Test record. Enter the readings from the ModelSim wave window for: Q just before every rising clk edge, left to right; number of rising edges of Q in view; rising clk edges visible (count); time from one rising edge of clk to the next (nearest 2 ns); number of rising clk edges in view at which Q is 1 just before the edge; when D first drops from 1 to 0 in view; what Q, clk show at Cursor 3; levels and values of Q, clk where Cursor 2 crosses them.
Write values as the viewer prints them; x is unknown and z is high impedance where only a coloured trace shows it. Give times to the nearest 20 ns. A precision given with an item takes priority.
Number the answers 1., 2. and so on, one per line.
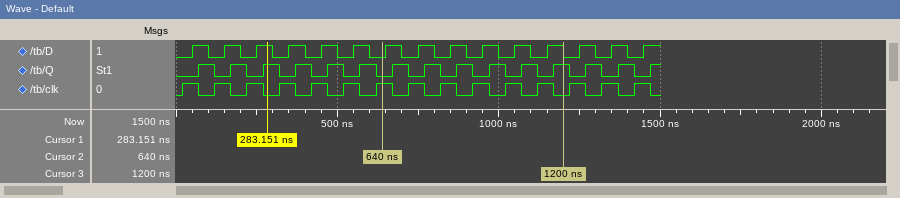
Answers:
1. 0 1 1 1 1 1 1 1 1 1 1 1 1 1 1
2. 15
3. 15
4. 100 ns
5. 14
6. 100 ns
7. Q=1, clk=0
8. Q=0, clk=1
